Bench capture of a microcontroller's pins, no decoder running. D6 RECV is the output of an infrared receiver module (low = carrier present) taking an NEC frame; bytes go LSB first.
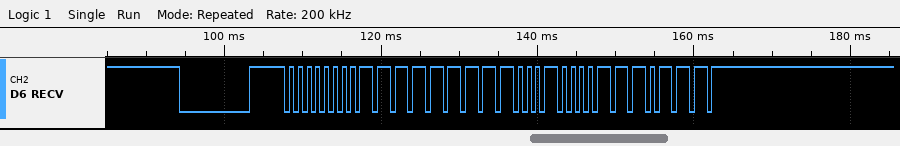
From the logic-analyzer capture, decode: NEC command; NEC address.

0x11
0x00
